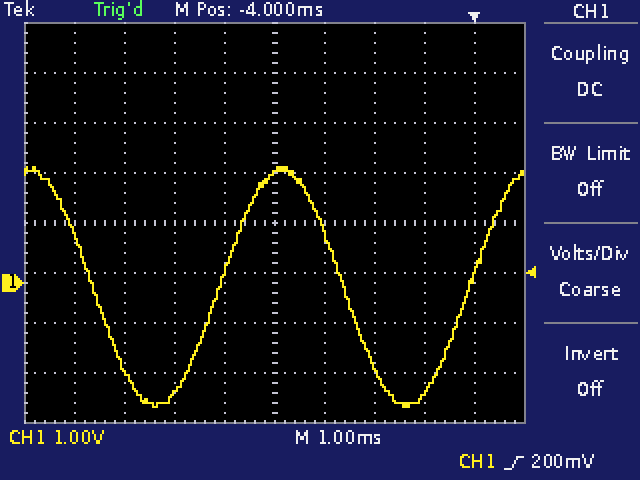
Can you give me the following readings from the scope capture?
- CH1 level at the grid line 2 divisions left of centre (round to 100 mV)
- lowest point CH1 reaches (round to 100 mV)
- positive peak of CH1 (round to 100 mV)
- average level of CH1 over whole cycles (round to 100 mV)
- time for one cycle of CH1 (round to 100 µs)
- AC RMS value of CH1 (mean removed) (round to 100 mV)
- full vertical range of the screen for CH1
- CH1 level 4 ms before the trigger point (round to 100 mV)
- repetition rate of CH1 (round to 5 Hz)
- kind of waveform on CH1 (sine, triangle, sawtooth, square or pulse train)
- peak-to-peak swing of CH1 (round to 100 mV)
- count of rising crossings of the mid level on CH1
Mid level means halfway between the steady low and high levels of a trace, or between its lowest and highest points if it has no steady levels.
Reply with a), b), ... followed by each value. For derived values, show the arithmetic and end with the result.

a) -2.2 V
b) -2.5 V
c) 2.3 V
d) (2.3 V + (-2.5 V)) / 2 ≈ -100 mV
e) 5.0 ms
f) 4.8 V / (2√2) ≈ 1.7 V
g) 8 V
h) 2.2 V
i) 1 / 5.0 ms ≈ 200 Hz
j) sine
k) 2.3 V − (-2.5 V) = 4.8 V
l) 2
